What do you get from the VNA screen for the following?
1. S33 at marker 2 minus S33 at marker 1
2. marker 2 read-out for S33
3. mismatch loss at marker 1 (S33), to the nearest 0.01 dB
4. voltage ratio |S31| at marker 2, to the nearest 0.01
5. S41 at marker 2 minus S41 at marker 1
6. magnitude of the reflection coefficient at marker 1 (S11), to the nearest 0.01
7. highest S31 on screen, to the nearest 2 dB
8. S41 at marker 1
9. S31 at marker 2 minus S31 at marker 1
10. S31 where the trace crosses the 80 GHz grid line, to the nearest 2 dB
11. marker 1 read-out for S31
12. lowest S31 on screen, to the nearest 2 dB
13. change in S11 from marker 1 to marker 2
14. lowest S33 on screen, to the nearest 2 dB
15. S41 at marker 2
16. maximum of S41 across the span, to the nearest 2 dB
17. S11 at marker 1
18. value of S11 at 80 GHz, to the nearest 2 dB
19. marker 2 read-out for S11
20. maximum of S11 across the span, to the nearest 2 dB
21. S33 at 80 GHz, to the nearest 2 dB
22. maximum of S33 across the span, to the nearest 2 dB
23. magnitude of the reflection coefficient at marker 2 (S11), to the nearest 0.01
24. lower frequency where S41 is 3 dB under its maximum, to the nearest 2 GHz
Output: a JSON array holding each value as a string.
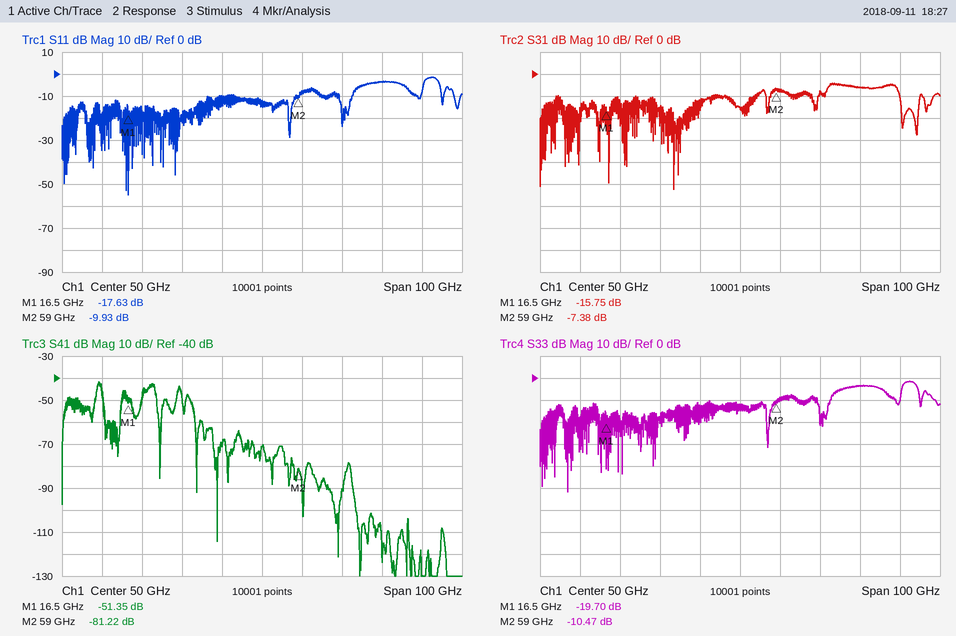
["9.23 dB", "-10.47 dB", "0.05 dB", "0.43", "-29.87 dB", "0.13", "-4 dB", "-51.35 dB", "8.37 dB", "-6 dB", "-15.75 dB", "-52 dB", "7.70 dB", "-52 dB", "-81.22 dB", "-42 dB", "-17.63 dB", "-4 dB", "-9.93 dB", "-2 dB", "-4 dB", "-2 dB", "0.32", "8 GHz"]
